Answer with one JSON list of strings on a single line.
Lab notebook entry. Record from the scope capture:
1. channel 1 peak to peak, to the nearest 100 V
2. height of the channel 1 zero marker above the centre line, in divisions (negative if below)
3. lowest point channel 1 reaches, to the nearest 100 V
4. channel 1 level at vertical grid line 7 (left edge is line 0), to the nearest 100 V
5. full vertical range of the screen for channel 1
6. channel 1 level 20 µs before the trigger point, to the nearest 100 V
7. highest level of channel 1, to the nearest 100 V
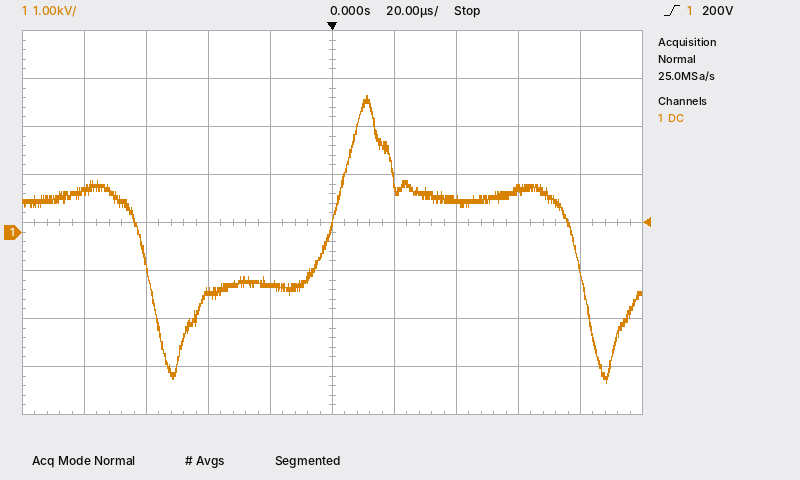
["6.0 kV", "-0.2 div", "-3.2 kV", "700 V", "8 kV", "-1.1 kV", "2.8 kV"]
